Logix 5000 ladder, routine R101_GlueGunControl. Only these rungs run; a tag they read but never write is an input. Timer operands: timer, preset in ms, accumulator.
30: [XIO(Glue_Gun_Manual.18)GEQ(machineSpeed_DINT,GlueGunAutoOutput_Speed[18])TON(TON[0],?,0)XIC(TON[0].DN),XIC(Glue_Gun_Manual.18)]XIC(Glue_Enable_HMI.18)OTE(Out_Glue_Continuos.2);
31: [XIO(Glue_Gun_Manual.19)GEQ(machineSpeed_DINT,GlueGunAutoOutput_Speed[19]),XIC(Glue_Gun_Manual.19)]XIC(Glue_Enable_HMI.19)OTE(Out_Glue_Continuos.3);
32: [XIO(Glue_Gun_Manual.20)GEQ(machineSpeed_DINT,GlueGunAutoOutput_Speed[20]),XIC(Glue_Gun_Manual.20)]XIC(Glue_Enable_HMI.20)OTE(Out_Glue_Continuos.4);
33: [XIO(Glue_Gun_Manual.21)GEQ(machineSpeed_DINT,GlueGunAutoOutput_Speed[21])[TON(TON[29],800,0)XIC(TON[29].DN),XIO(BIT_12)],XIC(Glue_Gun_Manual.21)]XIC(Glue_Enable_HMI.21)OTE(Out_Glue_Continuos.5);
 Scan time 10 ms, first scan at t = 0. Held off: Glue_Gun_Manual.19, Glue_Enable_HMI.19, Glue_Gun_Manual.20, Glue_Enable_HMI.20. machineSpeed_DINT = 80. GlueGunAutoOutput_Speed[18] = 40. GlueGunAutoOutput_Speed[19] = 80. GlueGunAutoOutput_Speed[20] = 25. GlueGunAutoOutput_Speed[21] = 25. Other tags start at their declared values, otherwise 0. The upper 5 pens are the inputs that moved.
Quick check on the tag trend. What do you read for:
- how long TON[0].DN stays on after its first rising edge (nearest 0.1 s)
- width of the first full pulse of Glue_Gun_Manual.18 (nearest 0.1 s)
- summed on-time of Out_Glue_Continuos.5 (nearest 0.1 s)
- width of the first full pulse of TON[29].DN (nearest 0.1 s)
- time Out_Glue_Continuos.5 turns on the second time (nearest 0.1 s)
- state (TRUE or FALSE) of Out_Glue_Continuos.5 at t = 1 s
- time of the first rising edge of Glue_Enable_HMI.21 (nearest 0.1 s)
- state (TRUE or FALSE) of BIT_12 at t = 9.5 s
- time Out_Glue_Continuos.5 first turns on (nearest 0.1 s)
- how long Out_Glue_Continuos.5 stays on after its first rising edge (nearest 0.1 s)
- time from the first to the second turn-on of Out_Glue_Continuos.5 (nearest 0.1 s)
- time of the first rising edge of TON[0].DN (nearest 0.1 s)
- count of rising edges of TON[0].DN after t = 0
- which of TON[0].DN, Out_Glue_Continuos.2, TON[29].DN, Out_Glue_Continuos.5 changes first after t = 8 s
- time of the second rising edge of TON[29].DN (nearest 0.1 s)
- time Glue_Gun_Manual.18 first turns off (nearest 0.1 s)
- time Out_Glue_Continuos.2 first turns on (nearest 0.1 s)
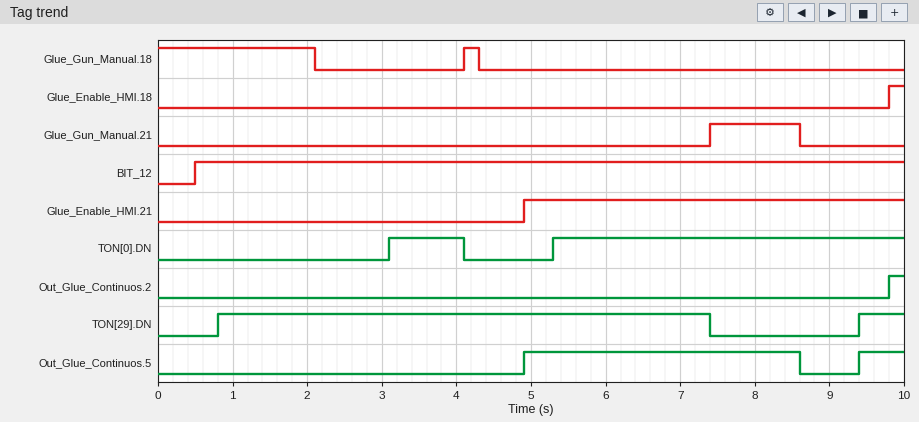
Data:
1.0 s
0.2 s
4.3 s
6.6 s
9.4 s
FALSE
4.9 s
TRUE
4.9 s
3.7 s
4.5 s
3.1 s
2
Out_Glue_Continuos.5
9.4 s
2.1 s
9.8 s
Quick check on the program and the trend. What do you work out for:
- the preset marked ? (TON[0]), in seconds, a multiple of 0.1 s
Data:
1.0 s
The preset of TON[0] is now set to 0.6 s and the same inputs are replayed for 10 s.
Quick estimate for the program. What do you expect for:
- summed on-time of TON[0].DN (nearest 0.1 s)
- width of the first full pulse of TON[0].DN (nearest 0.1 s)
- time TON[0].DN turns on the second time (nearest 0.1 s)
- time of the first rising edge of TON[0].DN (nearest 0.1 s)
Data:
6.5 s
1.4 s
4.9 s
2.7 s
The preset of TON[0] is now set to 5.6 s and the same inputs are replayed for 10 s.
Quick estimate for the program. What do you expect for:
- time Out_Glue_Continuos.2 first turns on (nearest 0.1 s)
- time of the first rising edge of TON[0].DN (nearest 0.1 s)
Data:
9.9 s
9.9 s
